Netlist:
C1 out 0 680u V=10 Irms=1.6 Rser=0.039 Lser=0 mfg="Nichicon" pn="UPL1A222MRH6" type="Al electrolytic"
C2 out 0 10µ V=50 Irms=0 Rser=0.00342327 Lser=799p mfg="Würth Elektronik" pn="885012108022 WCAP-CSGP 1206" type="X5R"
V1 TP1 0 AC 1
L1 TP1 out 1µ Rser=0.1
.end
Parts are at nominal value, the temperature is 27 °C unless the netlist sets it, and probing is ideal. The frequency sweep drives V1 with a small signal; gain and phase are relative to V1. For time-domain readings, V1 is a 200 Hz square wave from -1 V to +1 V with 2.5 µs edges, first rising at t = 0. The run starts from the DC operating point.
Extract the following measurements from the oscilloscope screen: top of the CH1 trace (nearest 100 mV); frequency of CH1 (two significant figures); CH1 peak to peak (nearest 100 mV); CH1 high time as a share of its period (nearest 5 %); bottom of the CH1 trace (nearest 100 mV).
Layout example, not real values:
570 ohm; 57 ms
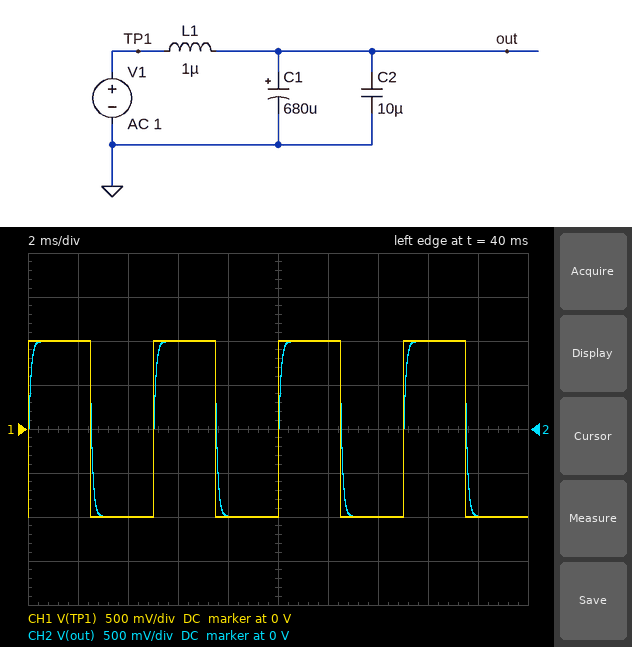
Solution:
1.0 V; 200 Hz; 2.0 V; 50 %; -1.0 V
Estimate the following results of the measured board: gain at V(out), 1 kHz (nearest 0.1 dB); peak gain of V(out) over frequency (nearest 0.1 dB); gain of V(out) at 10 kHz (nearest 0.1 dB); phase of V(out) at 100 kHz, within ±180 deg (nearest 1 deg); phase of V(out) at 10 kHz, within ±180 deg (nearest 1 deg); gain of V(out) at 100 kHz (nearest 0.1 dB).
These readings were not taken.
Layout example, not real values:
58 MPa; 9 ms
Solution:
-1.0 dB; 0 dB; -10.1 dB; -95 deg; -48 deg; -24.6 dB
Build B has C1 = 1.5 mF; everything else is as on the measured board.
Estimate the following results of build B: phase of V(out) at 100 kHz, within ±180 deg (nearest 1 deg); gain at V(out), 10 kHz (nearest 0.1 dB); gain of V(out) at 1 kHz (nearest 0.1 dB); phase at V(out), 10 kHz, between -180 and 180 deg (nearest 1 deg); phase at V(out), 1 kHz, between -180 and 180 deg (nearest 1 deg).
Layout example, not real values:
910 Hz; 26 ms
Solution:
-93 deg; -11.3 dB; -3.6 dB; -37 deg; -34 deg
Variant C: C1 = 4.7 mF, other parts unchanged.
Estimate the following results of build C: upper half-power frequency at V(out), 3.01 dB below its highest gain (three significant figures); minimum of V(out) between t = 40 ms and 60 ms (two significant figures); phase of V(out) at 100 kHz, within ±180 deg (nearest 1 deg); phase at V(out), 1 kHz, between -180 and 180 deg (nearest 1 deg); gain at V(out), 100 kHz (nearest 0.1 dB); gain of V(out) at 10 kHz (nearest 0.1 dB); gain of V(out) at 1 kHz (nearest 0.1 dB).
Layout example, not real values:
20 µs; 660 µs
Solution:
269 Hz; -970 mV; -92 deg; -30 deg; -24.5 dB; -11.7 dB; -8.8 dB
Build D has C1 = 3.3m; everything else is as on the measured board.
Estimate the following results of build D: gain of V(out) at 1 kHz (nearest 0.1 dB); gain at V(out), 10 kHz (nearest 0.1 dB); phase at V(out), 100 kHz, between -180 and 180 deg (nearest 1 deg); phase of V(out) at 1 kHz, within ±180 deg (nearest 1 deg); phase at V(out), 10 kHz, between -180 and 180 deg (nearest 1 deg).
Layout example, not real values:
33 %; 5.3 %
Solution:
-7.4 dB; -11.7 dB; -92 deg; -34 deg; -31 deg
